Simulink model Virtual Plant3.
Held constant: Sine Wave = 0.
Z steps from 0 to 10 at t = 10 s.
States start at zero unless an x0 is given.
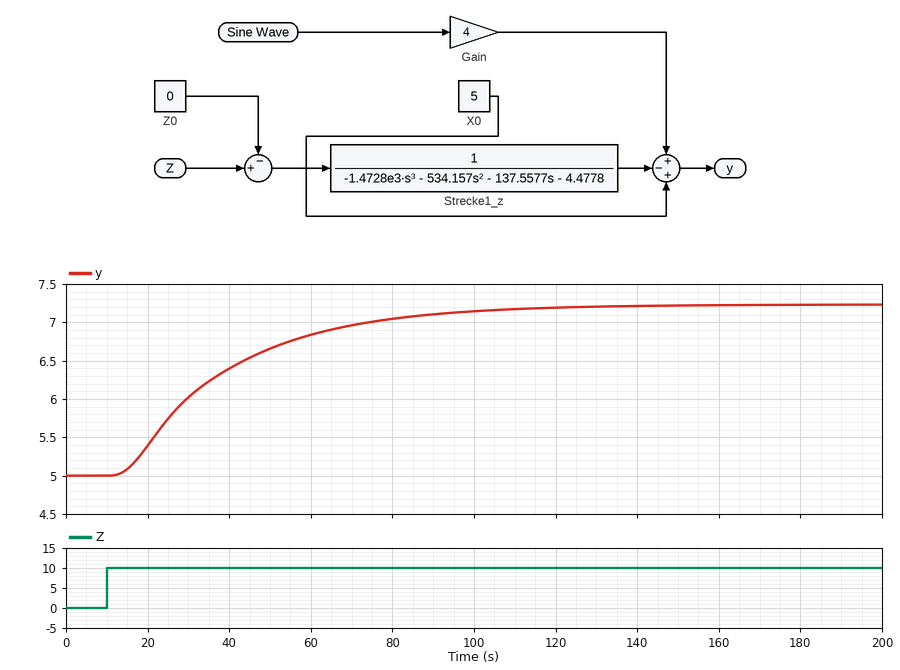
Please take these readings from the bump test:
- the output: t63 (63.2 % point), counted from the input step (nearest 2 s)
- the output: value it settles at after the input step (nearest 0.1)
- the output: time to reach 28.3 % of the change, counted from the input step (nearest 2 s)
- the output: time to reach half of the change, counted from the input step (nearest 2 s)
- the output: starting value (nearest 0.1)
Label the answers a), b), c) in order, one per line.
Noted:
a) 30 s
b) 7.2
c) 14 s
d) 22 s
e) 5.0
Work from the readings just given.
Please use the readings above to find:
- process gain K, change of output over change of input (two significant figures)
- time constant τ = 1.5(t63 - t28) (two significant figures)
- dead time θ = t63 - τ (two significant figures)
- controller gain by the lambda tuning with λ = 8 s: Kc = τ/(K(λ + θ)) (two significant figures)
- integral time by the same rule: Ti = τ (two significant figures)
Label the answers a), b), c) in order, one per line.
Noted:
a) 0.22
b) 24 s
c) 6.0 s
d) 7.8
e) 24 s
